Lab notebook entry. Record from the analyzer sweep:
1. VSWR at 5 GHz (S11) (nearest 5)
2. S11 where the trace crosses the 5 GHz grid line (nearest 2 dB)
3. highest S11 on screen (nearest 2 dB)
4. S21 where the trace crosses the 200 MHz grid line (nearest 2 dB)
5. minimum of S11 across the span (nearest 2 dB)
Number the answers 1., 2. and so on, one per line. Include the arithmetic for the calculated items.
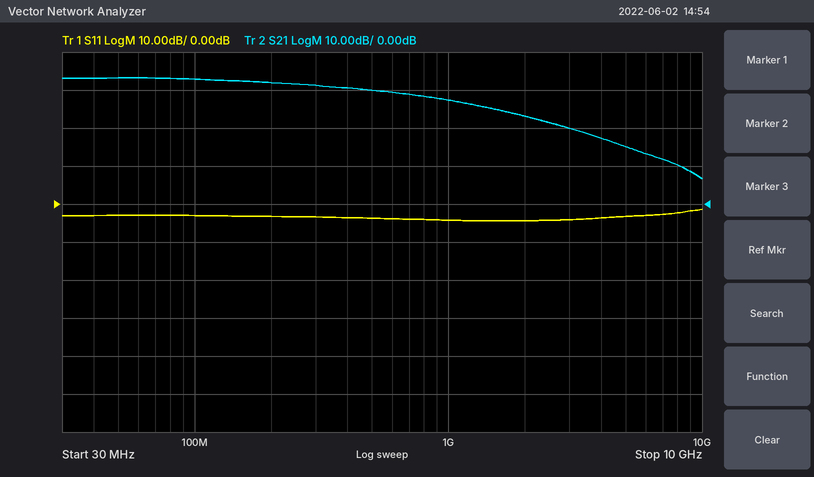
1. |Γ| = 10^(-4/20) = 0.6310; VSWR = (1 + 0.6310)/(1 − 0.6310) ≈ 4.42, so 5 to the nearest 5
2. -4 dB
3. -2 dB
4. 32 dB
5. -4 dB
